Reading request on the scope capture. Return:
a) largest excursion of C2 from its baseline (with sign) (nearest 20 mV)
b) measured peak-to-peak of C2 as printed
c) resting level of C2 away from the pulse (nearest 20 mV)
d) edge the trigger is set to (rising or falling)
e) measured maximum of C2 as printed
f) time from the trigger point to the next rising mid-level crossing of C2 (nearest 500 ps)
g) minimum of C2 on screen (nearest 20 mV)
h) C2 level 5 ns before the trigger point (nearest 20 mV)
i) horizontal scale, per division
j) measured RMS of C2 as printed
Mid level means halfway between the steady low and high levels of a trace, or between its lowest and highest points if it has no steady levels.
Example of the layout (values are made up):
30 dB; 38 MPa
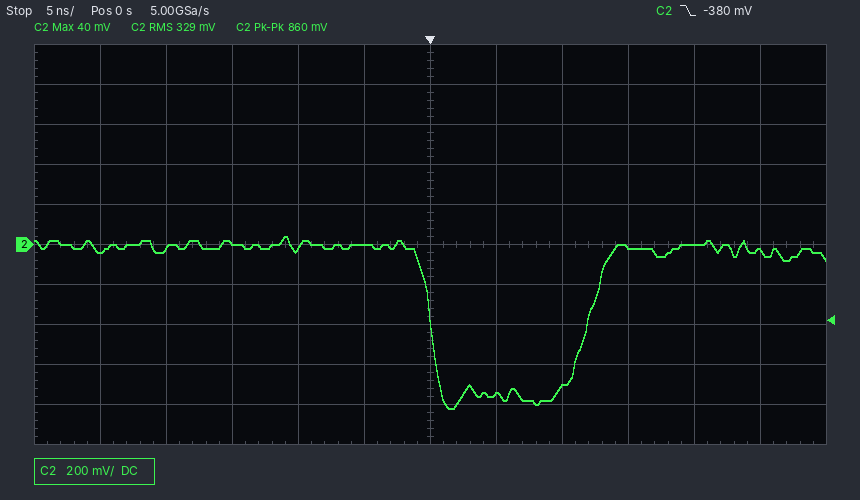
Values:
-800 mV; 860 mV; -20 mV; falling; 40 mV; 12.0 ns; -820 mV; 0 mV; 5 ns; 329 mV
